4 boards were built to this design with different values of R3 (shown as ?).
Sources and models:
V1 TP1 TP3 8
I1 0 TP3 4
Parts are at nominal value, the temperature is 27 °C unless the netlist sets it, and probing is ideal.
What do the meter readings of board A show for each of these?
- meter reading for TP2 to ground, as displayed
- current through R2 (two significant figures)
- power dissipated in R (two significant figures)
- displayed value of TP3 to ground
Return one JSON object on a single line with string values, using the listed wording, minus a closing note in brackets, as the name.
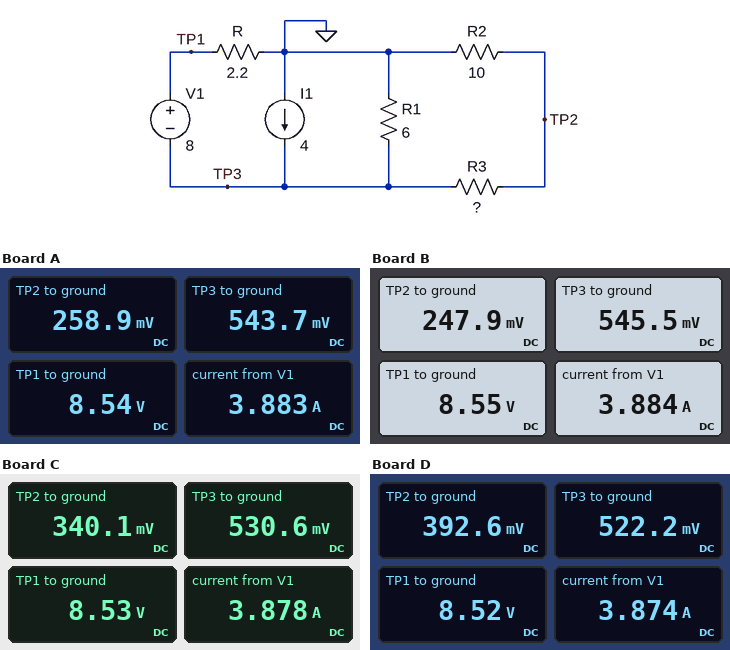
{"meter reading for TP2 to ground, as displayed": "258.9 mV", "current through R2": "26 mA", "power dissipated in R": "33 W", "displayed value of TP3 to ground": "543.7 mV"}
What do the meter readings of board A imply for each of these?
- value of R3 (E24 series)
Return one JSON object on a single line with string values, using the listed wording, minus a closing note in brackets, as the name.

{"value of R3": "11 Ω"}
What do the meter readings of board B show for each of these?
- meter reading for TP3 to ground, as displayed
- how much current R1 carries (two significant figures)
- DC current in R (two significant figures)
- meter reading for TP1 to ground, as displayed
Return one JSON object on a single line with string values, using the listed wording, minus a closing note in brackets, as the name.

{"meter reading for TP3 to ground, as displayed": "545.5 mV", "how much current R1 carries": "91 mA", "DC current in R": "3.9 A", "meter reading for TP1 to ground, as displayed": "8.55 V"}
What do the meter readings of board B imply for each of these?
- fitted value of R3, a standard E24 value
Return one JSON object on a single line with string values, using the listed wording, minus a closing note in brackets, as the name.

{"fitted value of R3, a standard E24 value": "12 Ω"}
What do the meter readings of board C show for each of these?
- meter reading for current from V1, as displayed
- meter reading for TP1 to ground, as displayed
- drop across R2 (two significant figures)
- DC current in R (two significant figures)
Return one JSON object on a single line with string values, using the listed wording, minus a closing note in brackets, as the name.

{"meter reading for current from V1, as displayed": "3.878 A", "meter reading for TP1 to ground, as displayed": "8.53 V", "drop across R2": "340 mV", "DC current in R": "3.9 A"}
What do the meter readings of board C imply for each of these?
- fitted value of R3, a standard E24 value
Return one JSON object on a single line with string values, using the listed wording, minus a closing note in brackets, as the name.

{"fitted value of R3, a standard E24 value": "5.6 Ω"}
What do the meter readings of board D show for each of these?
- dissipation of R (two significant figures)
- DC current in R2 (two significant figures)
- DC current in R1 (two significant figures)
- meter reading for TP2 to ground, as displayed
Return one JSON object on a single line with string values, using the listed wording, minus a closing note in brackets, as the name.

{"dissipation of R": "33 W", "DC current in R2": "39 mA", "DC current in R1": "87 mA", "meter reading for TP2 to ground, as displayed": "392.6 mV"}
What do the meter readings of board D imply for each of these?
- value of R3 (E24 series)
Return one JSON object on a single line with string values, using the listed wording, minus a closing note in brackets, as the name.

{"value of R3": "3.3 Ω"}
